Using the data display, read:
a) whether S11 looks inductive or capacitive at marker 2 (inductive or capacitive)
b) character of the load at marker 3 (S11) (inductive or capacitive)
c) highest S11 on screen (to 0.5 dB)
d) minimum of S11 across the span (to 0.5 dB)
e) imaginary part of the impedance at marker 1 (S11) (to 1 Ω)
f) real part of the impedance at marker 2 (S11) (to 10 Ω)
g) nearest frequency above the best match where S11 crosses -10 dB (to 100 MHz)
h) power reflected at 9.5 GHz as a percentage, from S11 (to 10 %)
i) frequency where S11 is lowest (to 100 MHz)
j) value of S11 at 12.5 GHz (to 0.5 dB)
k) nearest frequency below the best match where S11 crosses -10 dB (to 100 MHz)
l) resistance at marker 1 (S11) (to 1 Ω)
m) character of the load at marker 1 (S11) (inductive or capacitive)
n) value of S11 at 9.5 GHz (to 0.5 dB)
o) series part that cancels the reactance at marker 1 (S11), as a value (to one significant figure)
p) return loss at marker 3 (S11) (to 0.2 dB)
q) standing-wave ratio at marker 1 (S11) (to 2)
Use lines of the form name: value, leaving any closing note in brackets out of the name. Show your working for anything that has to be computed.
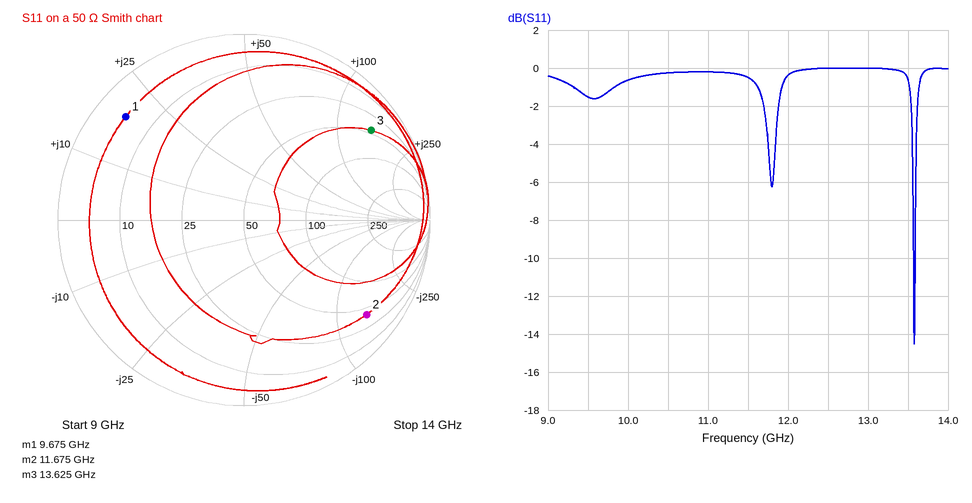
whether S11 looks inductive or capacitive at marker 2: capacitive
character of the load at marker 3 (S11): inductive
highest S11 on screen: 0.0 dB
minimum of S11 across the span: -14.5 dB
imaginary part of the impedance at marker 1 (S11): +19 Ω
real part of the impedance at marker 2 (S11): 40 Ω
nearest frequency above the best match where S11 crosses -10 dB: 13.6 GHz
power reflected at 9.5 GHz as a percentage, from S11: 10^(-1.5/10) ≈ 70.8 %, so 70 % to the nearest 10 %
frequency where S11 is lowest: 13.6 GHz
value of S11 at 12.5 GHz: 0.0 dB
nearest frequency below the best match where S11 crosses -10 dB: 13.6 GHz
resistance at marker 1 (S11): 5 Ω
character of the load at marker 1 (S11): inductive
value of S11 at 9.5 GHz: -1.5 dB
series part that cancels the reactance at marker 1 (S11), as a value: C = 1/(2π × 9.675 GHz × 19 Ω) ≈ 866 fF, so 900 fF to one significant figure
return loss at marker 3 (S11): 1.6 dB
standing-wave ratio at marker 1 (S11): 12
